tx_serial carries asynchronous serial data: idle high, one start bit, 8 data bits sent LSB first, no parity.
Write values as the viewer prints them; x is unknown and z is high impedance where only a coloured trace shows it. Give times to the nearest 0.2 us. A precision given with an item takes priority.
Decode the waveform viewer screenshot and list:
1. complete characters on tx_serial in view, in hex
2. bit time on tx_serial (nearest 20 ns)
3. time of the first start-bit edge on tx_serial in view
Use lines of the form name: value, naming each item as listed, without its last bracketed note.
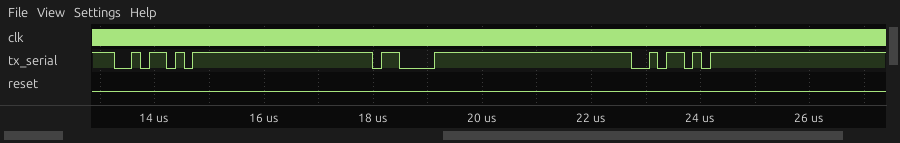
complete characters on tx_serial in view, in hex: 5A, C3, 5A
bit time on tx_serial: 160 ns
time of the first start-bit edge on tx_serial in view: 13.2 us
